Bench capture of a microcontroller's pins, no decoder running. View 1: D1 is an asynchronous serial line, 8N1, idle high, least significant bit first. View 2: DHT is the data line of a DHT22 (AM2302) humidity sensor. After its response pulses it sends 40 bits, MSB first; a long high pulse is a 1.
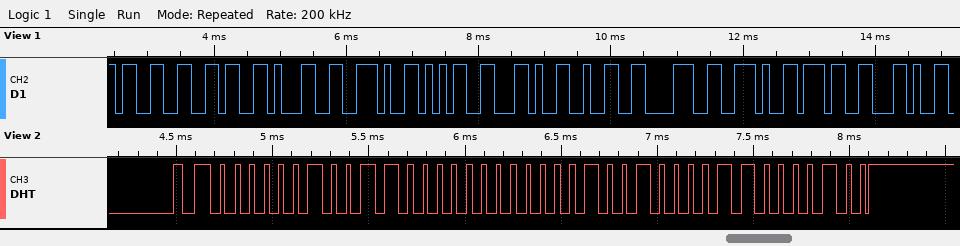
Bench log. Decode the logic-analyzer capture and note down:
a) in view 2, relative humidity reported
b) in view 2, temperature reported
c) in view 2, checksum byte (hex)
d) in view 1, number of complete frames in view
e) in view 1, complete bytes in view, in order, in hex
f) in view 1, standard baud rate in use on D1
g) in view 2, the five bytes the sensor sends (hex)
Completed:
60.8 %
28.9 °C
0x84
11
0x33 0x36 0x31 0x2E 0x35 0x2C 0x32 0x38 0x2E 0x37 0x2C
9600 baud
02 60 01 21 84
